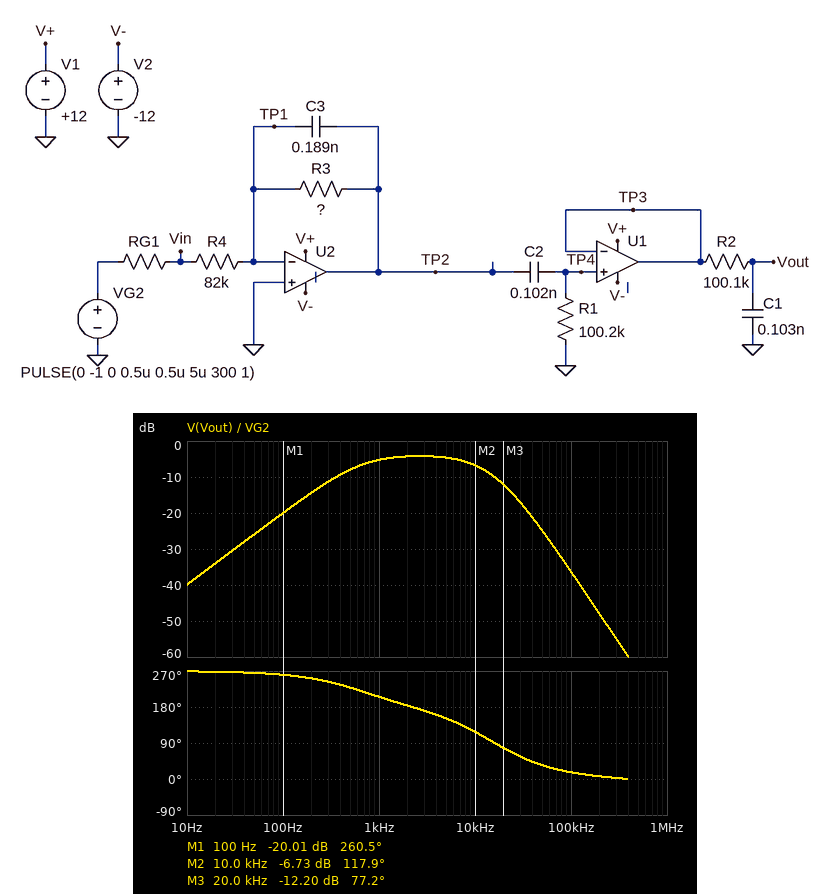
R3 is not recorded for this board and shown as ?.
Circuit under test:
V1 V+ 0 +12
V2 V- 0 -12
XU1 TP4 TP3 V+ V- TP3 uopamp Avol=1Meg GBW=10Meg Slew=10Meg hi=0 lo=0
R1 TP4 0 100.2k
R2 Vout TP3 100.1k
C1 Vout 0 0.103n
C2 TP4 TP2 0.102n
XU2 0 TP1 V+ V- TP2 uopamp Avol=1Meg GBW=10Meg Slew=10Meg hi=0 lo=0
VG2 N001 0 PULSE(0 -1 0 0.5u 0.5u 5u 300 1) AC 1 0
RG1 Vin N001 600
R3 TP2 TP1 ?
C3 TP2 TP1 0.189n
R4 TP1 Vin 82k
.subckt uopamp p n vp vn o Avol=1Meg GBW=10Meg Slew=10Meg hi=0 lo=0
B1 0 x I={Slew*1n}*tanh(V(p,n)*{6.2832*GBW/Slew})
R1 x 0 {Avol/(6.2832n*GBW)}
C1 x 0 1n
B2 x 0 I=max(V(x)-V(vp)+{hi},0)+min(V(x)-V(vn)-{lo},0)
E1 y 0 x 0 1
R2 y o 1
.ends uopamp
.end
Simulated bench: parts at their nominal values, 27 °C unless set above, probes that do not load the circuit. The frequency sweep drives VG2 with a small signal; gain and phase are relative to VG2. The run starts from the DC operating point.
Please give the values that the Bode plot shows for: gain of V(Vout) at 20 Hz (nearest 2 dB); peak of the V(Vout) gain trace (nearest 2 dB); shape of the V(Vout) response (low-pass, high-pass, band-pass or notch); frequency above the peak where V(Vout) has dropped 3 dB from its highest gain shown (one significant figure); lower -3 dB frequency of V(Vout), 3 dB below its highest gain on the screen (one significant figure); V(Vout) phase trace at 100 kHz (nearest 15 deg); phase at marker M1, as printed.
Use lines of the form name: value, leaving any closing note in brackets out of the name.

gain of V(Vout) at 20 Hz: -34 dB
peak of the V(Vout) gain trace: -4 dB
shape of the V(Vout) response: band-pass
frequency above the peak where V(Vout) has dropped 3 dB from its highest gain shown: 10 kHz
lower -3 dB frequency of V(Vout), 3 dB below its highest gain on the screen: 600 Hz
V(Vout) phase trace at 100 kHz: 15 deg
phase at marker M1, as printed: 260.5 deg
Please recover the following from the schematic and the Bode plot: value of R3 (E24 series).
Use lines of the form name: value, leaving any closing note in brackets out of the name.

value of R3: 1.3 MΩ
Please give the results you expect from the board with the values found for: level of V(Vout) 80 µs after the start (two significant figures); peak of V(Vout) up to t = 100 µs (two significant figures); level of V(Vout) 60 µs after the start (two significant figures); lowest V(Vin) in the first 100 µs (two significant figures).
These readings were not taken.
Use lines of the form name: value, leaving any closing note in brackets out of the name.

level of V(Vout) 80 µs after the start: -10 mV
peak of V(Vout) up to t = 100 µs: 120 mV
level of V(Vout) 60 µs after the start: -4.6 mV
lowest V(Vin) in the first 100 µs: -990 mV
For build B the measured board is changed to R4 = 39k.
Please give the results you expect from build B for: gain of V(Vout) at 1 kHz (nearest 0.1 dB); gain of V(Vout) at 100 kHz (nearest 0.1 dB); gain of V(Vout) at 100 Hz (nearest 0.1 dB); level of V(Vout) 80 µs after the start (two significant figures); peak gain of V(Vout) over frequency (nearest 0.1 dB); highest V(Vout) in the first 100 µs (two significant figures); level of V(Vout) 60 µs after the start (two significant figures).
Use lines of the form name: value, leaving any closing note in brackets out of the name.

gain of V(Vout) at 1 kHz: 1.1 dB
gain of V(Vout) at 100 kHz: -29.9 dB
gain of V(Vout) at 100 Hz: -13.6 dB
level of V(Vout) 80 µs after the start: -21 mV
peak gain of V(Vout) over frequency: 2.2 dB
highest V(Vout) in the first 100 µs: 260 mV
level of V(Vout) 60 µs after the start: -9.6 mV
